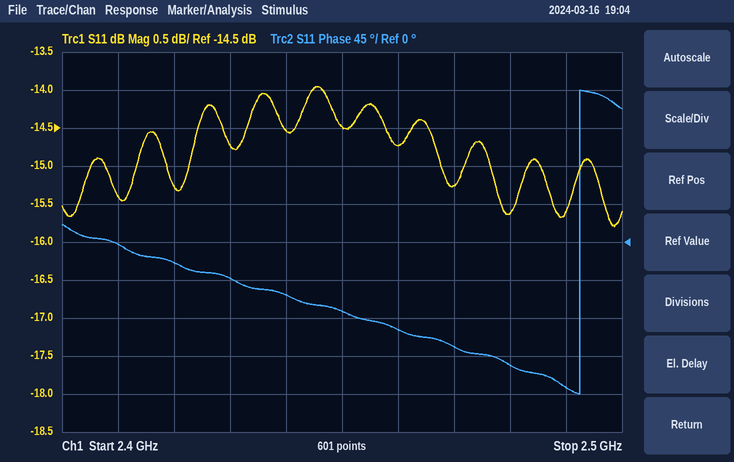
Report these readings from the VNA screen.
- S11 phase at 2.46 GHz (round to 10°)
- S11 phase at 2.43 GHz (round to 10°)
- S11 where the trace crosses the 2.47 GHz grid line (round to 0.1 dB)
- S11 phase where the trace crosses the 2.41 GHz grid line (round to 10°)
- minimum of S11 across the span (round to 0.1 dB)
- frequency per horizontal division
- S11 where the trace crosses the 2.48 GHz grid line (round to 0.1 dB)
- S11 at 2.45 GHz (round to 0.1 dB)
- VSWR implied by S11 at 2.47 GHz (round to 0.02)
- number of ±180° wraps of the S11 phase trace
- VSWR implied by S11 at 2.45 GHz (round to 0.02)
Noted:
-100°
-40°
-15.3 dB
0°
-15.8 dB
10 MHz
-15.6 dB
-14.5 dB
1.42
1
1.46
